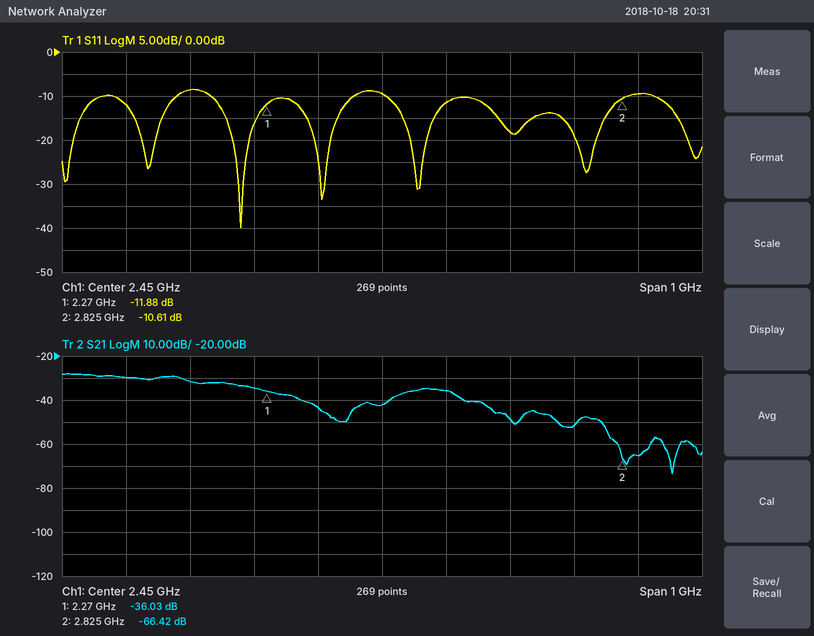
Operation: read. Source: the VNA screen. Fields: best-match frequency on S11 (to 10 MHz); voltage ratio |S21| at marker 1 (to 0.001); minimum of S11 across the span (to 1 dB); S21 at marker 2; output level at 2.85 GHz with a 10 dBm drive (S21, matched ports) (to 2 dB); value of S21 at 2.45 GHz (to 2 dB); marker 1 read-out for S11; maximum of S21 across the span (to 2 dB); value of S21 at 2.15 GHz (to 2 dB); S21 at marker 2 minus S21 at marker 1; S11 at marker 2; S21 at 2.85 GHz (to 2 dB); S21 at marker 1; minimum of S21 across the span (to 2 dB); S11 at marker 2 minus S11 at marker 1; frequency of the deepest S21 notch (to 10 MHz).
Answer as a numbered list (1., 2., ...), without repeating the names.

1. 2.23 GHz
2. 0.016
3. -40 dB
4. -66.42 dB
5. -56 dBm
6. -42 dB
7. -11.88 dB
8. -28 dB
9. -32 dB
10. -30.39 dB
11. -10.61 dB
12. -66 dB
13. -36.03 dB
14. -74 dB
15. 1.27 dB
16. 2.90 GHz
